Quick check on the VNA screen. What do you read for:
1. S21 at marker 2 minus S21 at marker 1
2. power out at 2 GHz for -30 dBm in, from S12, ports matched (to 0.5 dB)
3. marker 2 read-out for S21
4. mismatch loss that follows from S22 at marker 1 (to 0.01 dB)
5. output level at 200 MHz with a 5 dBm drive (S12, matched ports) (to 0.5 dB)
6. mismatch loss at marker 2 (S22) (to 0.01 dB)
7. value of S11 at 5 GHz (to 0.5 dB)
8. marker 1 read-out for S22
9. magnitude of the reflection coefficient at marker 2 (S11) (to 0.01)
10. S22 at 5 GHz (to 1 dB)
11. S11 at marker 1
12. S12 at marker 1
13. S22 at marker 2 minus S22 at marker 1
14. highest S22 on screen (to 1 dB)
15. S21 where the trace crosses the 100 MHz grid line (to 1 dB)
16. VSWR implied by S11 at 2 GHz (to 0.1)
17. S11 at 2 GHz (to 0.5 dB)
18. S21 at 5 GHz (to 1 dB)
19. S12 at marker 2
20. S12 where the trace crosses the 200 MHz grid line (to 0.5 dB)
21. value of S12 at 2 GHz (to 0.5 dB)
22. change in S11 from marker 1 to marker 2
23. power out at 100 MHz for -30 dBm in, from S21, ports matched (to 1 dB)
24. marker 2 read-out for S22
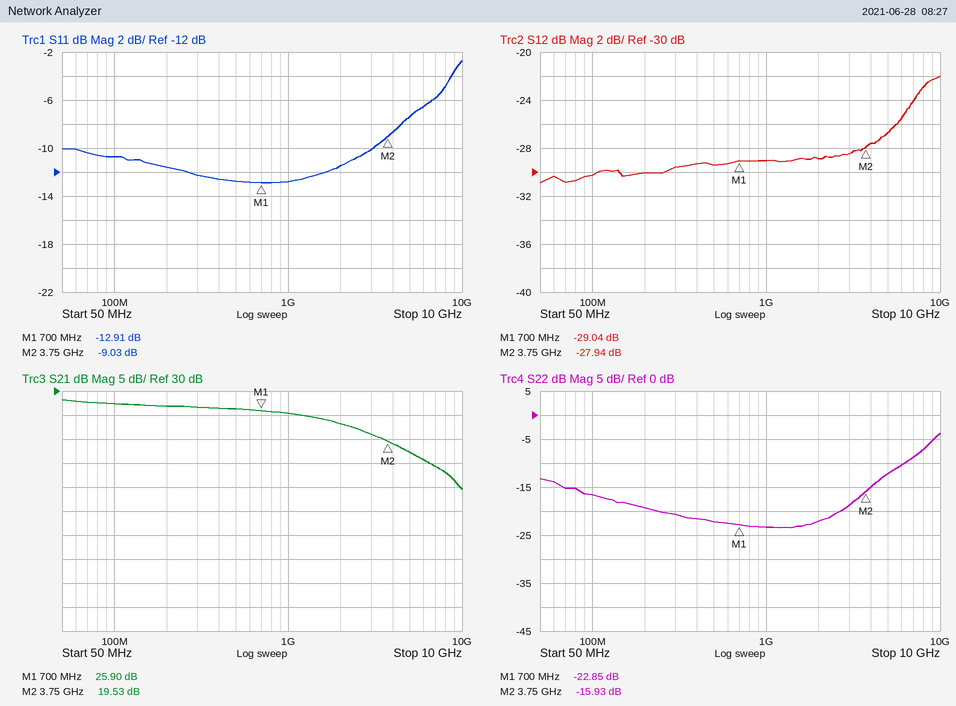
-6.37 dB
-59.0 dBm
19.53 dB
0.02 dB
-25.0 dBm
0.11 dB
-7.5 dB
-22.85 dB
0.35
-12 dB
-12.91 dB
-29.04 dB
6.92 dB
-4 dB
27 dB
1.7
-11.5 dB
17 dB
-27.94 dB
-30.0 dB
-29.0 dB
3.88 dB
-3 dBm
-15.93 dB
